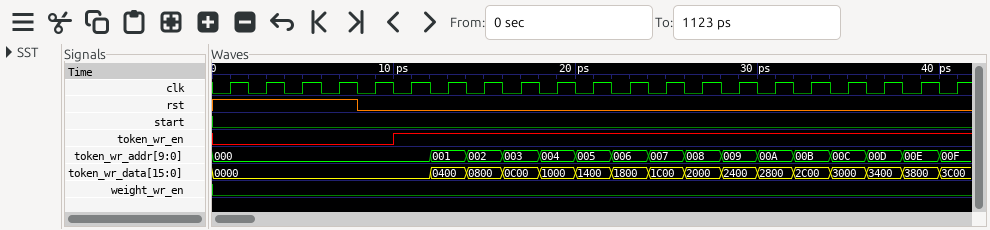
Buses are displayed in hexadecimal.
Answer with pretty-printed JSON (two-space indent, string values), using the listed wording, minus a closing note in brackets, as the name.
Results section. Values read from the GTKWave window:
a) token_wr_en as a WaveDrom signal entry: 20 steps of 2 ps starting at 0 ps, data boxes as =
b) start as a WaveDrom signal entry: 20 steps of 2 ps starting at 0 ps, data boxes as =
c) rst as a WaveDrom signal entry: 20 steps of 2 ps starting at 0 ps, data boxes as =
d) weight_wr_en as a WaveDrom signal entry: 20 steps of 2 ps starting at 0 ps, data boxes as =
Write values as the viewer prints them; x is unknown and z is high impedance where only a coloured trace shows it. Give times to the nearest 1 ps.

{
  "token_wr_en as a WaveDrom signal entry: 20 steps of 2 ps starting at 0 ps, data boxes as =": "{name: 'token_wr_en', wave: '0....1..............'}",
  "start as a WaveDrom signal entry: 20 steps of 2 ps starting at 0 ps, data boxes as =": "{name: 'start', wave: '0...................'}",
  "rst as a WaveDrom signal entry: 20 steps of 2 ps starting at 0 ps, data boxes as =": "{name: 'rst', wave: '1...0...............'}",
  "weight_wr_en as a WaveDrom signal entry: 20 steps of 2 ps starting at 0 ps, data boxes as =": "{name: 'weight_wr_en', wave: '0...................'}"
}
